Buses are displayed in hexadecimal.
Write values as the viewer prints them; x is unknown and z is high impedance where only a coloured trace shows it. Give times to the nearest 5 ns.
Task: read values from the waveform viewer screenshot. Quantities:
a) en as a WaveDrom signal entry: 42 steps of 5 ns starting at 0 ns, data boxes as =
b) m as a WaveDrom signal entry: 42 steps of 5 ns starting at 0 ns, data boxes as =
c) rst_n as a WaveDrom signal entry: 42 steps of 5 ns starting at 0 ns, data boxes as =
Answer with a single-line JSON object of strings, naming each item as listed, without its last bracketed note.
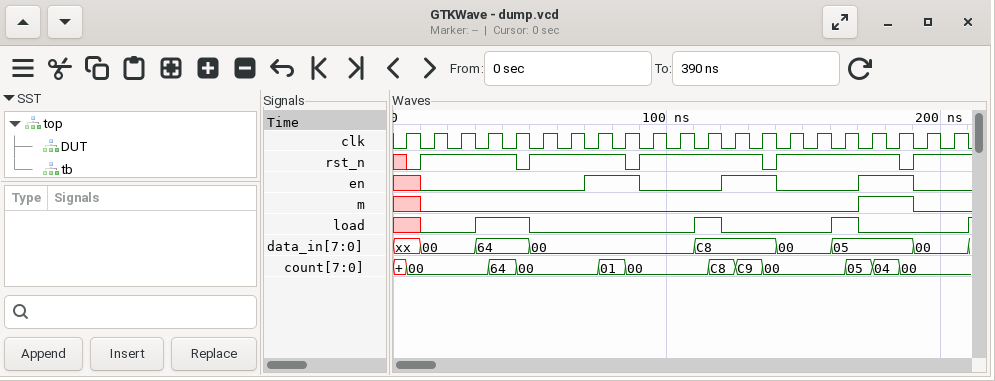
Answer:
{"en as a WaveDrom signal entry: 42 steps of 5 ns starting at 0 ns, data boxes as =": "{name: 'en', wave: 'x.0...........1...0.....1...0.....1...0...'}", "m as a WaveDrom signal entry: 42 steps of 5 ns starting at 0 ns, data boxes as =": "{name: 'm', wave: 'x.0...............................1...0...'}", "rst_n as a WaveDrom signal entry: 42 steps of 5 ns starting at 0 ns, data boxes as =": "{name: 'rst_n', wave: 'x01......01......01........01........01...'}"}
